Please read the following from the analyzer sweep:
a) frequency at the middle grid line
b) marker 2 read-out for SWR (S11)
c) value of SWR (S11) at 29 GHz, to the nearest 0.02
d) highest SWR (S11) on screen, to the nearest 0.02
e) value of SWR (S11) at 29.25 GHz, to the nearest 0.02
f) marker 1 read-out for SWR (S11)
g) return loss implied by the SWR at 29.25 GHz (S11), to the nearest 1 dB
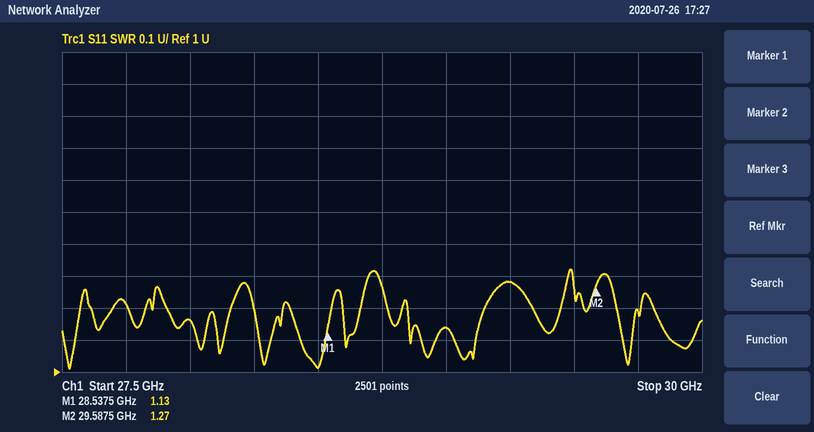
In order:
28.75 GHz
1.27
1.14
1.32
1.28
1.13
18 dB
